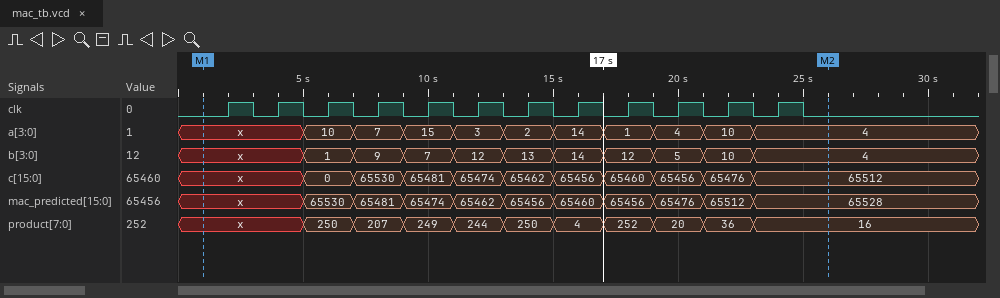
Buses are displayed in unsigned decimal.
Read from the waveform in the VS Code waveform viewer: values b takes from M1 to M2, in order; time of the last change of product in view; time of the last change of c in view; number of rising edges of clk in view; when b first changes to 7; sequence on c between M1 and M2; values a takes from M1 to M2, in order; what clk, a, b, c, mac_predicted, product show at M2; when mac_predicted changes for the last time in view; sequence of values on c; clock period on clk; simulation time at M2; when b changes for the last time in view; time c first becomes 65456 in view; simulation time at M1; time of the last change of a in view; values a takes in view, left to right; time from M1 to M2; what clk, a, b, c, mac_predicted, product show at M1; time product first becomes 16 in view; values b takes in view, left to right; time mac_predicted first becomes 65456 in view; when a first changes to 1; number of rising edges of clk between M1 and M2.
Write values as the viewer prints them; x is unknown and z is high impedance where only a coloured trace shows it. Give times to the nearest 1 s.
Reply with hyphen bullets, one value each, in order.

- x, 1, 9, 7, 12, 13, 14, 12, 5, 10, 4
- 23 s
- 23 s
- 12
- 9 s
- x, 0, 65530, 65481, 65474, 65462, 65456, 65460, 65456, 65476, 65512
- x, 10, 7, 15, 3, 2, 14, 1, 4, 10, 4
- clk=0, a=4, b=4, c=65512, mac_predicted=65528, product=16
- 23 s
- x, 0, 65530, 65481, 65474, 65462, 65456, 65460, 65456, 65476, 65512
- 2 s
- 26 s
- 23 s
- 15 s
- 1 s
- 23 s
- x, 10, 7, 15, 3, 2, 14, 1, 4, 10, 4
- 25 s
- clk=0, a=x, b=x, c=x, mac_predicted=x, product=x
- 23 s
- x, 1, 9, 7, 12, 13, 14, 12, 5, 10, 4
- 13 s
- 17 s
- 12
